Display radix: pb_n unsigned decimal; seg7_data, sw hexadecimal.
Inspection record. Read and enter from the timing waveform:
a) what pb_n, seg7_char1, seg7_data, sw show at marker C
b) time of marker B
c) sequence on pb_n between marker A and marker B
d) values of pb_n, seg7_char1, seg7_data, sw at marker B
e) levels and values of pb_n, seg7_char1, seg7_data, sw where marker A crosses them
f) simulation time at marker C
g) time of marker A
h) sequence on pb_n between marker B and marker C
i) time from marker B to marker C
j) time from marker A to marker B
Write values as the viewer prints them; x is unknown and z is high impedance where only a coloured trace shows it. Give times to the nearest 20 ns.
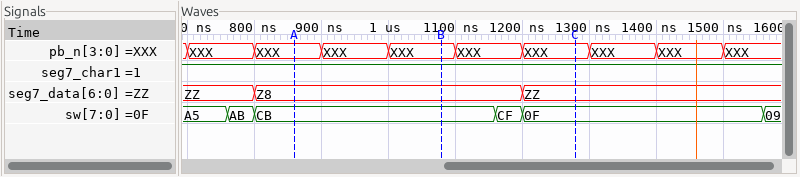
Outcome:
pb_n=XXX, seg7_char1=1, seg7_data=ZZ, sw=0F
1080 ns
XXX, XXX, XXX
pb_n=XXX, seg7_char1=1, seg7_data=Z8, sw=CB
pb_n=XXX, seg7_char1=1, seg7_data=Z8, sw=CB
1280 ns
860 ns
XXX, XXX, XXX
200 ns
220 ns
